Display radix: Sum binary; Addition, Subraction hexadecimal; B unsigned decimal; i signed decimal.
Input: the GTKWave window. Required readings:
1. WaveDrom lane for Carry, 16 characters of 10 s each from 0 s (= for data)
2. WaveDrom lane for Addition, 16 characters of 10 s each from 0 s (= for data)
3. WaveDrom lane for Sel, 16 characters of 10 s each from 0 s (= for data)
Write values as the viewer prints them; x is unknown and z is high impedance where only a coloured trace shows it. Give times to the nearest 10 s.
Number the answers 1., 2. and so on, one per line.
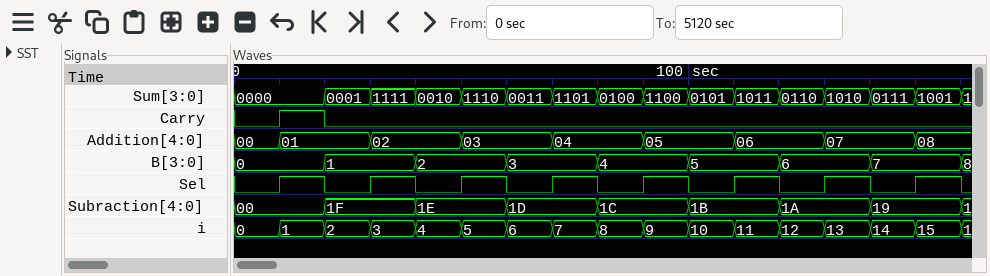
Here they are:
1. {name: 'Carry', wave: '010.............'}
2. {name: 'Addition', wave: '==.=.=.=.=.=.=.=', data: '00 01 02 03 04 05 06 07 08'}
3. {name: 'Sel', wave: '0101010101010101'}
